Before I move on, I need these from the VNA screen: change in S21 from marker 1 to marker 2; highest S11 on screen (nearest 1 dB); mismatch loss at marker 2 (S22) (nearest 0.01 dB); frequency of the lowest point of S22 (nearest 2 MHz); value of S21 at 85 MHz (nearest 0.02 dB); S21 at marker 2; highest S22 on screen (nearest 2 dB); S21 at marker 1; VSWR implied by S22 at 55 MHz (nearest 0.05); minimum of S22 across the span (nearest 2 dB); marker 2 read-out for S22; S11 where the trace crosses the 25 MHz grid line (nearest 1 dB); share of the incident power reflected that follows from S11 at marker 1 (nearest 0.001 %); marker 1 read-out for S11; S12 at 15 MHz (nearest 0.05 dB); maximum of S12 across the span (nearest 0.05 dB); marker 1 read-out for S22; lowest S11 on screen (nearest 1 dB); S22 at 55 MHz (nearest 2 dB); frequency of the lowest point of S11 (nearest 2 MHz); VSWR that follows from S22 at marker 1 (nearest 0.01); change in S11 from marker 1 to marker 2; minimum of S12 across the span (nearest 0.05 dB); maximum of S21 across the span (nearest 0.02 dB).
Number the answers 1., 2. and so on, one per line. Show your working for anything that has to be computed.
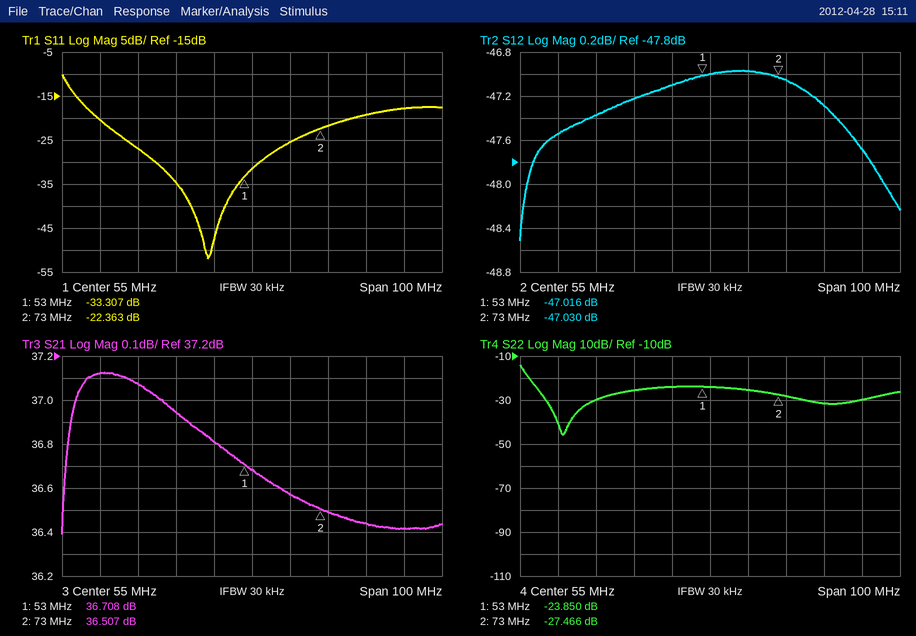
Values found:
1. 36.507 − (36.708) = -0.201 dB
2. -10 dB
3. −10 log10(1 − 10^(-27.466/10)) ≈ 0.01 dB
4. 16 MHz
5. 36.44 dB
6. 36.507 dB
7. -14 dB
8. 36.708 dB
9. |Γ| = 10^(-24/20) = 0.0631; VSWR = (1 + 0.0631)/(1 − 0.0631) ≈ 1.13, so 1.15 to the nearest 0.05
10. -46 dB
11. -27.466 dB
12. -27 dB
13. 10^(-33.307/10) ≈ 0.047 %
14. -33.307 dB
15. -47.55 dB
16. -46.95 dB
17. -23.850 dB
18. -52 dB
19. -24 dB
20. 44 MHz
21. (1 + 0.0642)/(1 − 0.0642) ≈ 1.14
22. -22.363 − (-33.307) = 10.944 dB
23. -48.50 dB
24. 37.12 dB
